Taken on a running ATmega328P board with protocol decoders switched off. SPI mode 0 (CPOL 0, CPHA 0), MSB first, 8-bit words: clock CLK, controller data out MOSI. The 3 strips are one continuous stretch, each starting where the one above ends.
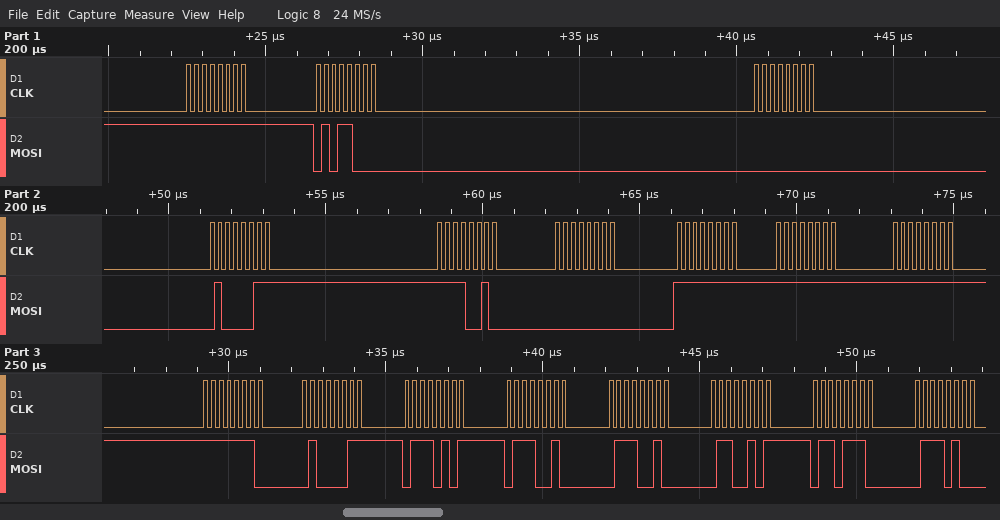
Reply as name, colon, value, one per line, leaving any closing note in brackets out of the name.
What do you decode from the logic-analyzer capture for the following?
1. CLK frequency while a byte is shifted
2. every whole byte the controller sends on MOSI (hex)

CLK frequency while a byte is shifted: 4 MHz
every whole byte the controller sends on MOSI: 0xFF 0x58 0x00 0x43 0xF2 0x00 0xFF 0xFF 0xFF 0xFE 0x43 0x75 0x72 0x72 0x65 0x6E 0x74
